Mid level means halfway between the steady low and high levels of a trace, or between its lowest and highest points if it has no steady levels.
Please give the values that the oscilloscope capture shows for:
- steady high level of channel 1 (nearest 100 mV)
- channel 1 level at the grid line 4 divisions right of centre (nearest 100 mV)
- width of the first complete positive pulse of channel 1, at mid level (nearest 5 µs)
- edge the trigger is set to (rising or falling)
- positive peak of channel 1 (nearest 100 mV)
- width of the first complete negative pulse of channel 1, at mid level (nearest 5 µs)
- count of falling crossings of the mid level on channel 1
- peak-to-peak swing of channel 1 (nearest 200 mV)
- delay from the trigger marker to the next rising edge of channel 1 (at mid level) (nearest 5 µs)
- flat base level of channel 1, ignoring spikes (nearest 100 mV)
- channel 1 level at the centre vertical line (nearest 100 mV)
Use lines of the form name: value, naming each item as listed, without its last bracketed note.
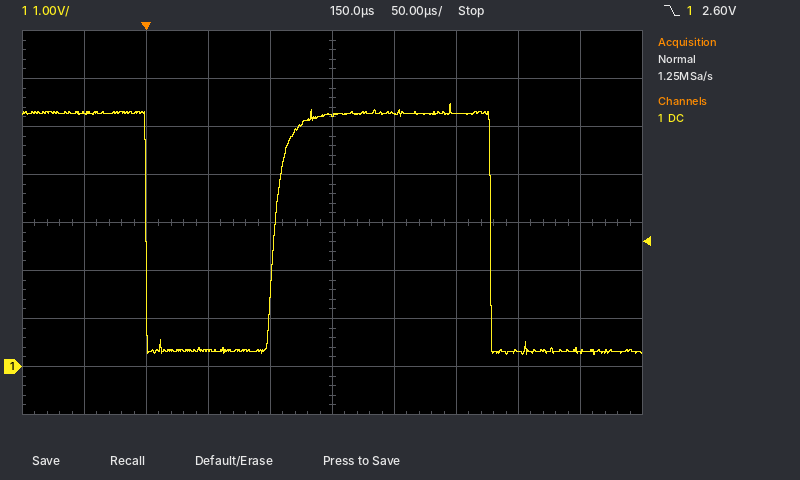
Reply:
steady high level of channel 1: 5.3 V
channel 1 level at the grid line 4 divisions right of centre: 300 mV
width of the first complete positive pulse of channel 1, at mid level: 175 µs
edge the trigger is set to: falling
positive peak of channel 1: 5.5 V
width of the first complete negative pulse of channel 1, at mid level: 105 µs
count of falling crossings of the mid level on channel 1: 2
peak-to-peak swing of channel 1: 5.2 V
delay from the trigger marker to the next rising edge of channel 1 (at mid level): 105 µs
flat base level of channel 1, ignoring spikes: 300 mV
channel 1 level at the centre vertical line: 5.2 V
